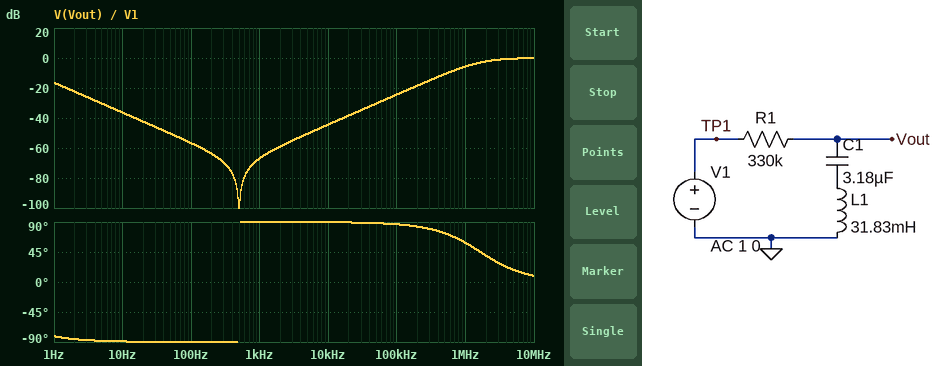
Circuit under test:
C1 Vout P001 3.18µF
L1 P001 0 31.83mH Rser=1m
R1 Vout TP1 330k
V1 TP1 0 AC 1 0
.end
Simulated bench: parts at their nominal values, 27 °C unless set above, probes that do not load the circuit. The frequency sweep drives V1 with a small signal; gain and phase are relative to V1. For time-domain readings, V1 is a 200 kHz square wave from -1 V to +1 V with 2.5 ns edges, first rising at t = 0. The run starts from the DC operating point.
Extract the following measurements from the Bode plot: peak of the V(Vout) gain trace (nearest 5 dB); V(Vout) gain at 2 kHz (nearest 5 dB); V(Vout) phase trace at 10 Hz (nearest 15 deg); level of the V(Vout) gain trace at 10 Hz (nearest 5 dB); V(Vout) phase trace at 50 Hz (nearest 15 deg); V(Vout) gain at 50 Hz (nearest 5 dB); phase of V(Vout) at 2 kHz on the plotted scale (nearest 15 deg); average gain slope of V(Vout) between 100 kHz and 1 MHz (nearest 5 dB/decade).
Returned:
0 dB
-60 dB
-90 deg
-35 dB
-90 deg
-50 dB
90 deg
20 dB/decade
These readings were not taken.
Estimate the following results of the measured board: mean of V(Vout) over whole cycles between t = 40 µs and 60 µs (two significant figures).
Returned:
-1.0 V
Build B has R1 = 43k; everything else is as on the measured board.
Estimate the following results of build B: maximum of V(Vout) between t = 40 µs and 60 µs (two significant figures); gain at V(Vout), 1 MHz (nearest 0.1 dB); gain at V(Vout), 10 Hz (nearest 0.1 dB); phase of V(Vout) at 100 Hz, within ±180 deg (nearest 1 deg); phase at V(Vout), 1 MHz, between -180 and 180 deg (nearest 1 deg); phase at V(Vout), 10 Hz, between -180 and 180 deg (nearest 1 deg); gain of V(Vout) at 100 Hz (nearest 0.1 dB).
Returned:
930 mV
-0.2 dB
-18.7 dB
-89 deg
12 deg
-83 deg
-39.0 dB
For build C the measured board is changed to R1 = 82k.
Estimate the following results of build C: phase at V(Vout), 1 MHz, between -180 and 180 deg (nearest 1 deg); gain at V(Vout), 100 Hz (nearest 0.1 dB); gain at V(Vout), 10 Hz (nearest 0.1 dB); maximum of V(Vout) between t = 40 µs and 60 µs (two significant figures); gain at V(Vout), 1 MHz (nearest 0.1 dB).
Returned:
22 deg
-44.6 dB
-24.3 dB
990 mV
-0.7 dB
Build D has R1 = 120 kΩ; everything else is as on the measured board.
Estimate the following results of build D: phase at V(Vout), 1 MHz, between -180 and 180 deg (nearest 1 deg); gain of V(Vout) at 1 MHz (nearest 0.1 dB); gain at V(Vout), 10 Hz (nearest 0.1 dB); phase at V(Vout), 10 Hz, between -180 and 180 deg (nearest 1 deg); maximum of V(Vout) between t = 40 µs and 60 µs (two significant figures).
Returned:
31 deg
-1.3 dB
-27.6 dB
-88 deg
990 mV
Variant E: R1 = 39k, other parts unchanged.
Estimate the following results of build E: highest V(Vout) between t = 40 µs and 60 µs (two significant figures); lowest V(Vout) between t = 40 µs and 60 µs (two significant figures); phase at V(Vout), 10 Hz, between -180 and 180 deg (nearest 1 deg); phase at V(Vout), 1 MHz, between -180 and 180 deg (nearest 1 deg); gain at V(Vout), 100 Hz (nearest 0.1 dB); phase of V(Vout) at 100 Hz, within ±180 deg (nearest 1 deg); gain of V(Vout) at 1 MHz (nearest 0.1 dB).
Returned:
910 mV
-2.9 V
-83 deg
11 deg
-38.2 dB
-89 deg
-0.2 dB
